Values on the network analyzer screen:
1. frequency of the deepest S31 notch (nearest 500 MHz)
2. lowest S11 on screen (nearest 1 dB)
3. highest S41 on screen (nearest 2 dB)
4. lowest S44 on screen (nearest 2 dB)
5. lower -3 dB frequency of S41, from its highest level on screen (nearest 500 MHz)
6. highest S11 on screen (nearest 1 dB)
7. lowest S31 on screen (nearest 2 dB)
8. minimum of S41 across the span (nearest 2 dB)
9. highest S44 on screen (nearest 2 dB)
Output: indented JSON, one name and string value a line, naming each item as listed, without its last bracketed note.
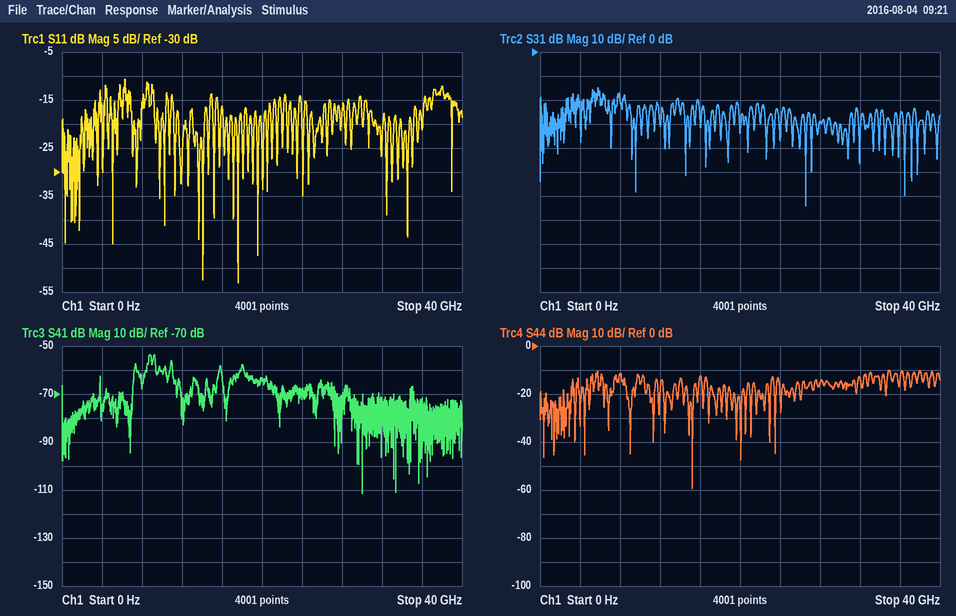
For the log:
{
  "frequency of the deepest S31 notch": "26.5 GHz",
  "lowest S11 on screen": "-53 dB",
  "highest S41 on screen": "-54 dB",
  "lowest S44 on screen": "-60 dB",
  "lower -3 dB frequency of S41, from its highest level on screen": "8.5 GHz",
  "highest S11 on screen": "-11 dB",
  "lowest S31 on screen": "-64 dB",
  "minimum of S41 across the span": "-112 dB",
  "highest S44 on screen": "-10 dB"
}
